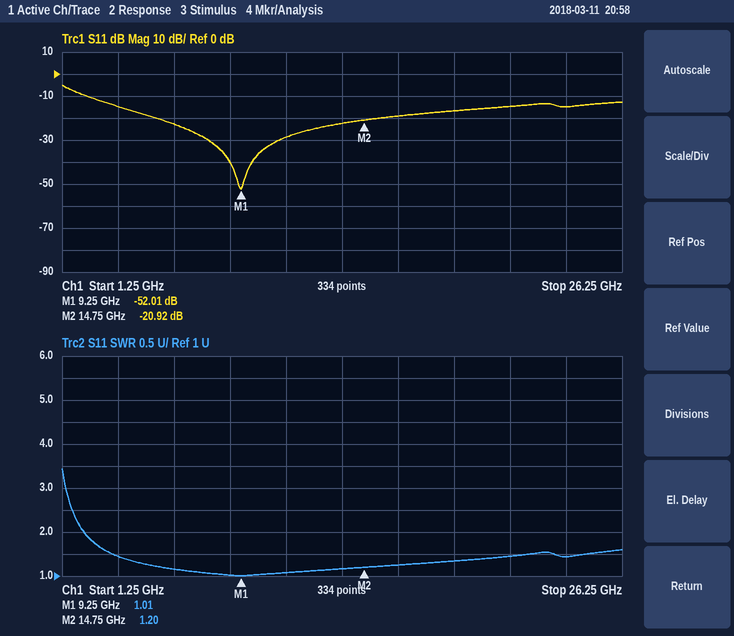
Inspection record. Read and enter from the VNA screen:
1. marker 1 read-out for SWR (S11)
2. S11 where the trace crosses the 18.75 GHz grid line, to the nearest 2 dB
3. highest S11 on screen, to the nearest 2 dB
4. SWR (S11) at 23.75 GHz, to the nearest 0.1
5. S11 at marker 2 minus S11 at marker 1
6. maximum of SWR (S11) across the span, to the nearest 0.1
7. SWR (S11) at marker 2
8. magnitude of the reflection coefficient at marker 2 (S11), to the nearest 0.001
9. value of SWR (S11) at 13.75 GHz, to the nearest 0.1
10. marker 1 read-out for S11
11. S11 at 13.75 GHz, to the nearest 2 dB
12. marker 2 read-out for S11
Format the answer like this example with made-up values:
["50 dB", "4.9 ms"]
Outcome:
["1.01", "-16 dB", "-6 dB", "1.4", "31.09 dB", "3.4", "1.20", "0.090", "1.2", "-52.01 dB", "-22 dB", "-20.92 dB"]
